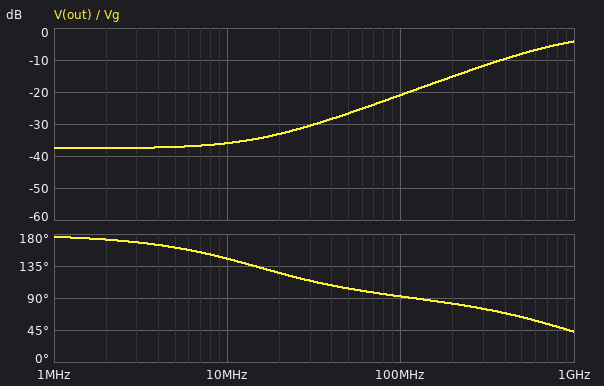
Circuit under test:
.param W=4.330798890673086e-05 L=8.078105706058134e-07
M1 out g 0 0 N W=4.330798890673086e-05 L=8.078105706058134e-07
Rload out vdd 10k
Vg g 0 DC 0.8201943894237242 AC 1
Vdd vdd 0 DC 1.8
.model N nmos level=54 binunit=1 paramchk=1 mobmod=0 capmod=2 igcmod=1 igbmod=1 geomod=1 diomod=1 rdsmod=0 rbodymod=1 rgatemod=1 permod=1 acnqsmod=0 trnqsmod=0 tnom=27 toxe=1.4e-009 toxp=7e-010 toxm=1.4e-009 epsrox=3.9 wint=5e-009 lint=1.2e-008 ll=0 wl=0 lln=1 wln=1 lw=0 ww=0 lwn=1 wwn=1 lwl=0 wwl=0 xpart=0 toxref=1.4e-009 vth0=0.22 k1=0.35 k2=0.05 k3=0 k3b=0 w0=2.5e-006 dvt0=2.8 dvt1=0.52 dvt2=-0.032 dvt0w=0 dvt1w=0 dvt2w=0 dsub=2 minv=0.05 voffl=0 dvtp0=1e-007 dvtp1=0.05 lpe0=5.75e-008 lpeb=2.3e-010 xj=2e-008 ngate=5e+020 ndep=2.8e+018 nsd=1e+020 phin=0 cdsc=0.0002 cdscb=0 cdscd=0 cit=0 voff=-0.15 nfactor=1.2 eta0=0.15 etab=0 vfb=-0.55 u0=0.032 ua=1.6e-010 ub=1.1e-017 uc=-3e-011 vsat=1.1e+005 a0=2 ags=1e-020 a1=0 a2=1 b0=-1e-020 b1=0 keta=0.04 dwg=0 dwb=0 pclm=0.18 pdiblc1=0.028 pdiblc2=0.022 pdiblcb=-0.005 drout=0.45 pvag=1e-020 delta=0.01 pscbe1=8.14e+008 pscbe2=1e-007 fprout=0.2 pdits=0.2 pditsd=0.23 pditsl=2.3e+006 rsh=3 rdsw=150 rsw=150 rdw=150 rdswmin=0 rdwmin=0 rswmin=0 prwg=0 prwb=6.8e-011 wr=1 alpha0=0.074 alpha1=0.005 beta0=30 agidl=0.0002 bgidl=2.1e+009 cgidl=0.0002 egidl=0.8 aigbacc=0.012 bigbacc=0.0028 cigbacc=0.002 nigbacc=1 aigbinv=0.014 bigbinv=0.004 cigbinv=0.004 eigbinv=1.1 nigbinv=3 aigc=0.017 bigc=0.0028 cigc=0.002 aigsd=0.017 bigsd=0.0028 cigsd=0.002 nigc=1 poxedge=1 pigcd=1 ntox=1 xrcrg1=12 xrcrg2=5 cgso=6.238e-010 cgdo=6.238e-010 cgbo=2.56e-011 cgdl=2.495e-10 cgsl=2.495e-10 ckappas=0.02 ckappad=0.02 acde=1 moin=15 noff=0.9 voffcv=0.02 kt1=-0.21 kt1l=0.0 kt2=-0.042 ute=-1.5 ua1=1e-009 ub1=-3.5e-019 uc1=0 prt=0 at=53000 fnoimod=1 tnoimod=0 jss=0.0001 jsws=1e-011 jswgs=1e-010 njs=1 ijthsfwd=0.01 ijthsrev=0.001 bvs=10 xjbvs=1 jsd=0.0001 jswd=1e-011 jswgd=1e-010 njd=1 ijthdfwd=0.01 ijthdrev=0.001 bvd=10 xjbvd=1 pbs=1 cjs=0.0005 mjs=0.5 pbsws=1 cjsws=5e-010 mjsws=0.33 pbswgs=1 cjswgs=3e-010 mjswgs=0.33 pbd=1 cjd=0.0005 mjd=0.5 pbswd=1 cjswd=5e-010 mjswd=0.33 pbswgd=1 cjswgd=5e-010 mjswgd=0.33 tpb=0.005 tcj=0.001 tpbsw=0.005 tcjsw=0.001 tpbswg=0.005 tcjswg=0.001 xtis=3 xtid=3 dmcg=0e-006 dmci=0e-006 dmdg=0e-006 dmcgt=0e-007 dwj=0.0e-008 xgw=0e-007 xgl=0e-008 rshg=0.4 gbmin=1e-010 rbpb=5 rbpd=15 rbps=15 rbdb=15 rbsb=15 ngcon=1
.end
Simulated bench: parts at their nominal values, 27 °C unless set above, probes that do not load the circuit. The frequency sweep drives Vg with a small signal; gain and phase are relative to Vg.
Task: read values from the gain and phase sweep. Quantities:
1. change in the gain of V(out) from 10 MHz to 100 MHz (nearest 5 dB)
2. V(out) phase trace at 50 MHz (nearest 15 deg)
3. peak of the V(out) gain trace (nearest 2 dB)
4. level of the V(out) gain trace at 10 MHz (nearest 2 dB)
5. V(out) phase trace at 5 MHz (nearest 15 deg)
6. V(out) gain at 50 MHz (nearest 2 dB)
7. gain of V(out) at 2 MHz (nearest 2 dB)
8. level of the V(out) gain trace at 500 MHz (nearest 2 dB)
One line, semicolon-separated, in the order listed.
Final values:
15 dB; 105 deg; -4 dB; -36 dB; 165 deg; -26 dB; -38 dB; -8 dB
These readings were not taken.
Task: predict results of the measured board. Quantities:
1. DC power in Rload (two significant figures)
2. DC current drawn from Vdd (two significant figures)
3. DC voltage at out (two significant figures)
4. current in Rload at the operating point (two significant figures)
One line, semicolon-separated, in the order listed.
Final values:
310 µW; 180 µA; 35 mV; 180 µA
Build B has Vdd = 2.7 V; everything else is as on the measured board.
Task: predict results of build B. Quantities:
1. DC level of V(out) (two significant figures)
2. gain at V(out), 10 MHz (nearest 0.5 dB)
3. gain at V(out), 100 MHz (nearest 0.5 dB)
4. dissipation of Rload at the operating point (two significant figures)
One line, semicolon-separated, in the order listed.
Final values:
54 mV; -32.0 dB; -20.5 dB; 700 µW
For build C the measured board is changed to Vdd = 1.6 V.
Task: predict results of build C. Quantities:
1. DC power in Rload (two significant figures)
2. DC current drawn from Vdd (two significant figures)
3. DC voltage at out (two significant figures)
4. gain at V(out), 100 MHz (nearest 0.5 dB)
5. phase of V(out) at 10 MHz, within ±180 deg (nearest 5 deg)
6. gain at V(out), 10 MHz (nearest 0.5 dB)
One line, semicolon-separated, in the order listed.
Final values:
250 µW; 160 µA; 31 mV; -21.0 dB; 140 deg; -37.0 dB
